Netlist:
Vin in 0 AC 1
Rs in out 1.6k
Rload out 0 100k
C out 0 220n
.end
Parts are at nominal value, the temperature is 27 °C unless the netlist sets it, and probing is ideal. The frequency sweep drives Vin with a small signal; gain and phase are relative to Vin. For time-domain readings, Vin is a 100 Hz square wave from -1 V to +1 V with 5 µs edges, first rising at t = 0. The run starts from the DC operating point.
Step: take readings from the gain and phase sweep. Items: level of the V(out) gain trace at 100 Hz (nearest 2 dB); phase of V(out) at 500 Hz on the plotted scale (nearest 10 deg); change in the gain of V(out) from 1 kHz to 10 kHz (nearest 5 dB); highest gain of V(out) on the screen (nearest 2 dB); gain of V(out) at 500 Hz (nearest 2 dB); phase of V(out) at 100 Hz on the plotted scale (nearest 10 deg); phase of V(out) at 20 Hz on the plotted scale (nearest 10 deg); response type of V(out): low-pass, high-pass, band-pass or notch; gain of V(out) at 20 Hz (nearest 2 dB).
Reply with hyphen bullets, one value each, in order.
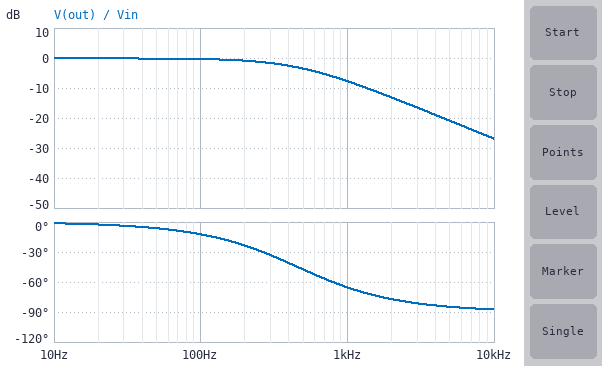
- 0 dB
- -50 deg
- -20 dB
- 0 dB
- -4 dB
- -10 deg
- 0 deg
- low-pass
- 0 dB
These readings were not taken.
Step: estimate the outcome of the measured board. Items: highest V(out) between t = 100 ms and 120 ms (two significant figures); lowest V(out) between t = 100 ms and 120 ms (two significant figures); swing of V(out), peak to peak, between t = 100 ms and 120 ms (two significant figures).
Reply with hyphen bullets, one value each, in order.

- 980 mV
- -980 mV
- 2.0 V
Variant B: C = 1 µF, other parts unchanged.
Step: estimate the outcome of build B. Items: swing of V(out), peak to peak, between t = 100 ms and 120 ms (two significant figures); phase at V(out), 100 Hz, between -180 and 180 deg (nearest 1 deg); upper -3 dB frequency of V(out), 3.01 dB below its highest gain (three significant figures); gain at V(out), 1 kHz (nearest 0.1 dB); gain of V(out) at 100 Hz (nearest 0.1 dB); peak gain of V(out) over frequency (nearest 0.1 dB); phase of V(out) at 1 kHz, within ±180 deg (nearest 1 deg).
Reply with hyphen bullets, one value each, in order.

- 1.8 V
- -45 deg
- 101 Hz
- -20.1 dB
- -3.1 dB
- -0.1 dB
- -84 deg
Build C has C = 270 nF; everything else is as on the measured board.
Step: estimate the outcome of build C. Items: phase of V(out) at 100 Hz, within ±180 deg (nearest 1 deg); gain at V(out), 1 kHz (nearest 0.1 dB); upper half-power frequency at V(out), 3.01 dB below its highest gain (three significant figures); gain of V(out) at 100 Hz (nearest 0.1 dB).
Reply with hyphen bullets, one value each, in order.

- -15 deg
- -9.2 dB
- 374 Hz
- -0.4 dB
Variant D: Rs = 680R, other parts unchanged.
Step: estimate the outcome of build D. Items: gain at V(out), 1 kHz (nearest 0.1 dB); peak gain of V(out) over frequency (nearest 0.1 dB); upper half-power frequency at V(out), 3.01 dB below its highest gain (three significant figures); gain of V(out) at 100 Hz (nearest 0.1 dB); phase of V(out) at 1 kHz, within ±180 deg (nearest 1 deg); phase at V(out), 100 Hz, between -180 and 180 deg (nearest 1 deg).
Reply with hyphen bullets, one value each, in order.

- -2.8 dB
- -0.1 dB
- 1.07 kHz
- -0.1 dB
- -43 deg
- -5 deg
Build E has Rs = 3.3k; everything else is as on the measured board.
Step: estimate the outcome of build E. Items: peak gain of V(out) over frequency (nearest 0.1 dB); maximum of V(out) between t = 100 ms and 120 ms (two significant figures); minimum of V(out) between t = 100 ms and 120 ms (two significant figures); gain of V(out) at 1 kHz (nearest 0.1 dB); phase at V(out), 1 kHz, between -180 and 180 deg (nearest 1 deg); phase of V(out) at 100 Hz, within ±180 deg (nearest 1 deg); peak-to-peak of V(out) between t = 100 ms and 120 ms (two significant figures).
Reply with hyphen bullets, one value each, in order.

- -0.3 dB
- 970 mV
- -970 mV
- -13.4 dB
- -77 deg
- -24 deg
- 1.9 V
